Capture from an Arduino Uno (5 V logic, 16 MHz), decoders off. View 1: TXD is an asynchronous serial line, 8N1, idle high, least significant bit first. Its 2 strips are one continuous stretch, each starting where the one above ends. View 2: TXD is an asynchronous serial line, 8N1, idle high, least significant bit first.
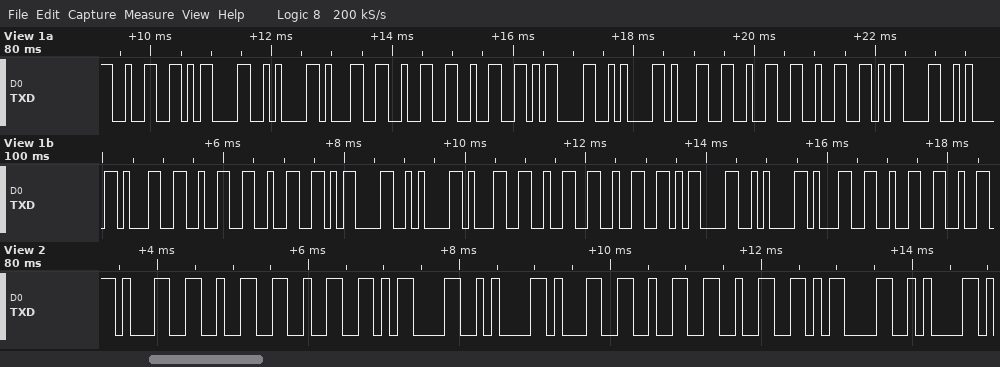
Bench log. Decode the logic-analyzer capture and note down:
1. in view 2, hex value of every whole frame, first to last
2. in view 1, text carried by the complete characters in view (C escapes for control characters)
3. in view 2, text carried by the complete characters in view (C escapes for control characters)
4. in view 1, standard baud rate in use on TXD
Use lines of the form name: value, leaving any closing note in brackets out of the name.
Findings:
in view 2, hex value of every whole frame, first to last: 31 32 32 0D 0A 31 32 32 0D 0A
in view 1, text carried by the complete characters in view: "2\r\n122\r\n122\r\n122\r\n122\r\n12"
in view 2, text carried by the complete characters in view: "122\r\n122\r\n"
in view 1, standard baud rate in use on TXD: 9600 baud
